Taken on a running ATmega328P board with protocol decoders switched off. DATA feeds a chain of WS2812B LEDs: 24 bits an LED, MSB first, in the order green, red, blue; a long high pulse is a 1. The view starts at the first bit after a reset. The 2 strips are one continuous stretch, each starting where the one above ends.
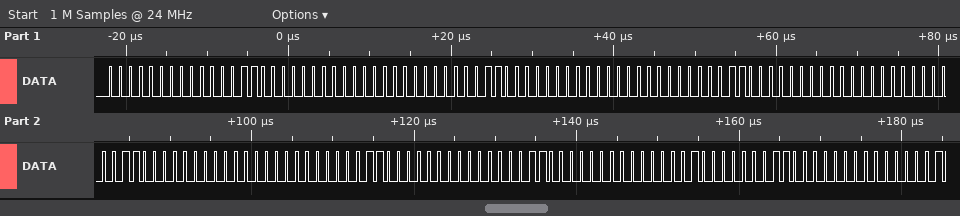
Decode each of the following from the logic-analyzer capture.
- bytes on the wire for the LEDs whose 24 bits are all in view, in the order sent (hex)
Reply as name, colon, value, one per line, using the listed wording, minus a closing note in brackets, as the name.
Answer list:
bytes on the wire for the LEDs whose 24 bits are all in view, in the order sent: 00 06 00 00 06 00 00 06 00 00 06 00 00 06 00 06 00 04
